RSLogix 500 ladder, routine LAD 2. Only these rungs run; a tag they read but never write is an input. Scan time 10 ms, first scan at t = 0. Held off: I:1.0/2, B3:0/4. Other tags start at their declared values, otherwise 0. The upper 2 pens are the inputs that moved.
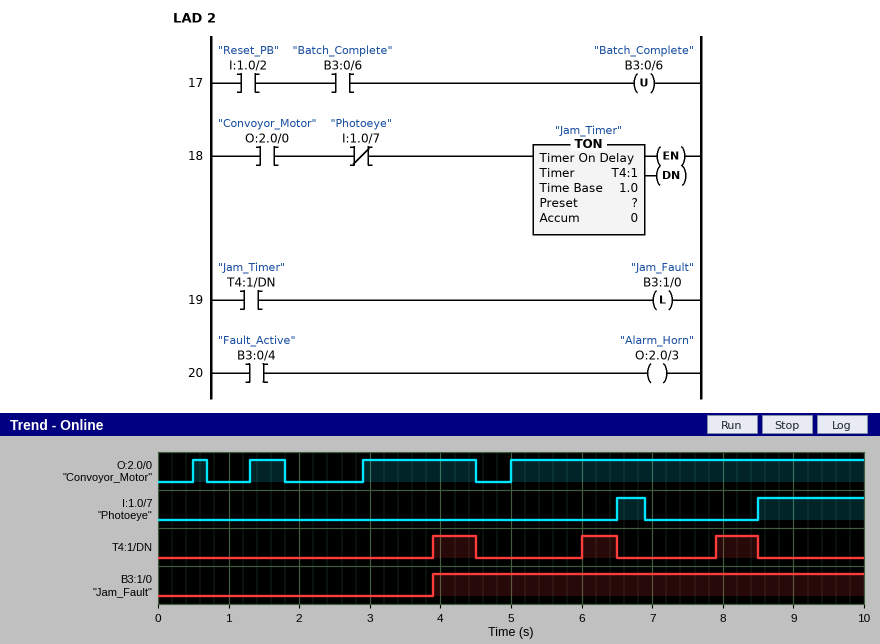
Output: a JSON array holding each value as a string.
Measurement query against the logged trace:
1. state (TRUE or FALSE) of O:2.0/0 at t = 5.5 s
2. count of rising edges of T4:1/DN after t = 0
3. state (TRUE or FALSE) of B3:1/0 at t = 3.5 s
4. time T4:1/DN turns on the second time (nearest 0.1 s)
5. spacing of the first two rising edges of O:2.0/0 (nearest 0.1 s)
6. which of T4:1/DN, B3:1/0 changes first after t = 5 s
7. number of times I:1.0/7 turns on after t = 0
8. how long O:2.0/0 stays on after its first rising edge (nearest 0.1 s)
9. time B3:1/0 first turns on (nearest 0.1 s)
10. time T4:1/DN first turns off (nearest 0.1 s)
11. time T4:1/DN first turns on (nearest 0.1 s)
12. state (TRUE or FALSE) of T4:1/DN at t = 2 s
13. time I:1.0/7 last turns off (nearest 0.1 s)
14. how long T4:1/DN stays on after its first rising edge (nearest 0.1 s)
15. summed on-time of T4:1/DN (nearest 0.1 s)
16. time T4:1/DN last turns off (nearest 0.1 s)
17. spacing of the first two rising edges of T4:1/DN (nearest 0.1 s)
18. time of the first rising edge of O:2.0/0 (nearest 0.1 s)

["TRUE", "3", "FALSE", "6.0 s", "0.8 s", "T4:1/DN", "2", "0.2 s", "3.9 s", "4.5 s", "3.9 s", "FALSE", "6.9 s", "0.6 s", "1.7 s", "8.5 s", "2.1 s", "0.5 s"]
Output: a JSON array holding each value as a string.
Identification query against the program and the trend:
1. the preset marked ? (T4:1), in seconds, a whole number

["1 s"]
